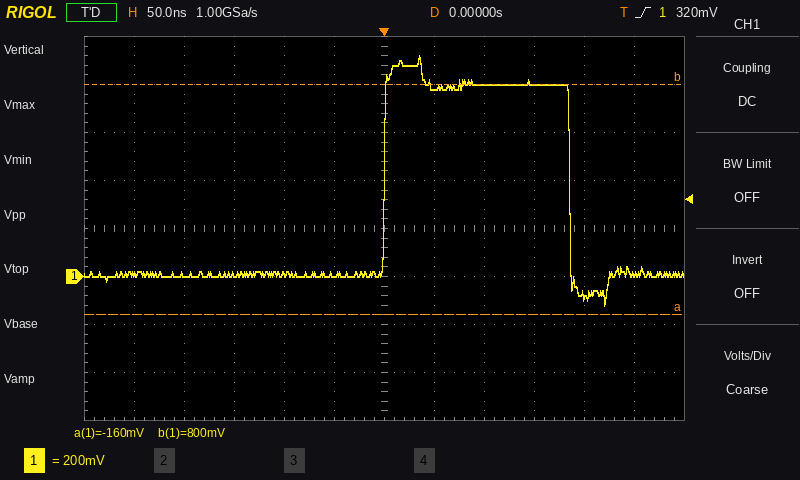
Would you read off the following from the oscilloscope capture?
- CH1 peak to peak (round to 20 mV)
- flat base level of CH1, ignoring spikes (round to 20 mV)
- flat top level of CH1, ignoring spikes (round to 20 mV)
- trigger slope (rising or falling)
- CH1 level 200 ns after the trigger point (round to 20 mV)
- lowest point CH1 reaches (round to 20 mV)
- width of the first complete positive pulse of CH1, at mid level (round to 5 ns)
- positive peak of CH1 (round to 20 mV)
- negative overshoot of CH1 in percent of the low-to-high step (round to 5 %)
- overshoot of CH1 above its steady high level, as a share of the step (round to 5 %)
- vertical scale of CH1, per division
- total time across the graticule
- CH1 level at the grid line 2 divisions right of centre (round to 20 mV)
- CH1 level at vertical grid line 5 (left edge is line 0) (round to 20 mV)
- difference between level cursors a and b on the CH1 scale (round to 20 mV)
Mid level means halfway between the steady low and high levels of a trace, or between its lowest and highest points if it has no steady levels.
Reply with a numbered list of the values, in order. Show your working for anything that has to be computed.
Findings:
1. 920 mV − (-120 mV) = 1.04 V
2. 0 mV
3. 800 mV
4. rising
5. -80 mV
6. -120 mV
7. 185 ns
8. 920 mV
9. 15 %
10. 15 %
11. 200 mV
12. 600 ns
13. 800 mV
14. 0 mV
15. 960 mV
